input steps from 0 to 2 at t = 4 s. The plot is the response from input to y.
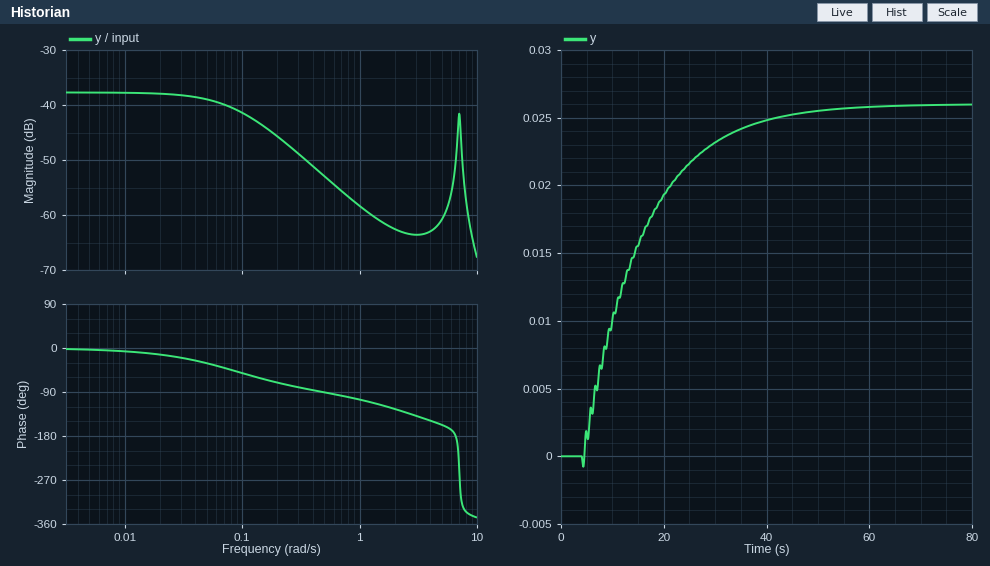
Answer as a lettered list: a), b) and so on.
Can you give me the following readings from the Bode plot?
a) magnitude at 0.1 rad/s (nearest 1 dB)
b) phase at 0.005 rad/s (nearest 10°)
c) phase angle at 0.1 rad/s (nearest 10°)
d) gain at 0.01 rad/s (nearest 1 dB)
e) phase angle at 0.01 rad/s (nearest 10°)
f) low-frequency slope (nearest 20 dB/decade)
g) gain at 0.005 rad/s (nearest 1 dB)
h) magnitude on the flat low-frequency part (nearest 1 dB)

a) -41 dB
b) 0°
c) -50°
d) -38 dB
e) -10°
f) 0 dB/decade
g) -38 dB
h) -38 dB
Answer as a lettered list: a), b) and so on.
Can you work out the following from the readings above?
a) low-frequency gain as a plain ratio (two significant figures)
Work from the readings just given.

a) 0.013
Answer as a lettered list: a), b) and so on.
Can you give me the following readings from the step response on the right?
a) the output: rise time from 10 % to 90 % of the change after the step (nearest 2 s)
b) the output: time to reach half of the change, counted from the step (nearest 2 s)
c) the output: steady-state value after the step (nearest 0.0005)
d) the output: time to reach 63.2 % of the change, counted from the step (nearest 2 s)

a) 26 s
b) 8 s
c) 0.0260
d) 12 s
